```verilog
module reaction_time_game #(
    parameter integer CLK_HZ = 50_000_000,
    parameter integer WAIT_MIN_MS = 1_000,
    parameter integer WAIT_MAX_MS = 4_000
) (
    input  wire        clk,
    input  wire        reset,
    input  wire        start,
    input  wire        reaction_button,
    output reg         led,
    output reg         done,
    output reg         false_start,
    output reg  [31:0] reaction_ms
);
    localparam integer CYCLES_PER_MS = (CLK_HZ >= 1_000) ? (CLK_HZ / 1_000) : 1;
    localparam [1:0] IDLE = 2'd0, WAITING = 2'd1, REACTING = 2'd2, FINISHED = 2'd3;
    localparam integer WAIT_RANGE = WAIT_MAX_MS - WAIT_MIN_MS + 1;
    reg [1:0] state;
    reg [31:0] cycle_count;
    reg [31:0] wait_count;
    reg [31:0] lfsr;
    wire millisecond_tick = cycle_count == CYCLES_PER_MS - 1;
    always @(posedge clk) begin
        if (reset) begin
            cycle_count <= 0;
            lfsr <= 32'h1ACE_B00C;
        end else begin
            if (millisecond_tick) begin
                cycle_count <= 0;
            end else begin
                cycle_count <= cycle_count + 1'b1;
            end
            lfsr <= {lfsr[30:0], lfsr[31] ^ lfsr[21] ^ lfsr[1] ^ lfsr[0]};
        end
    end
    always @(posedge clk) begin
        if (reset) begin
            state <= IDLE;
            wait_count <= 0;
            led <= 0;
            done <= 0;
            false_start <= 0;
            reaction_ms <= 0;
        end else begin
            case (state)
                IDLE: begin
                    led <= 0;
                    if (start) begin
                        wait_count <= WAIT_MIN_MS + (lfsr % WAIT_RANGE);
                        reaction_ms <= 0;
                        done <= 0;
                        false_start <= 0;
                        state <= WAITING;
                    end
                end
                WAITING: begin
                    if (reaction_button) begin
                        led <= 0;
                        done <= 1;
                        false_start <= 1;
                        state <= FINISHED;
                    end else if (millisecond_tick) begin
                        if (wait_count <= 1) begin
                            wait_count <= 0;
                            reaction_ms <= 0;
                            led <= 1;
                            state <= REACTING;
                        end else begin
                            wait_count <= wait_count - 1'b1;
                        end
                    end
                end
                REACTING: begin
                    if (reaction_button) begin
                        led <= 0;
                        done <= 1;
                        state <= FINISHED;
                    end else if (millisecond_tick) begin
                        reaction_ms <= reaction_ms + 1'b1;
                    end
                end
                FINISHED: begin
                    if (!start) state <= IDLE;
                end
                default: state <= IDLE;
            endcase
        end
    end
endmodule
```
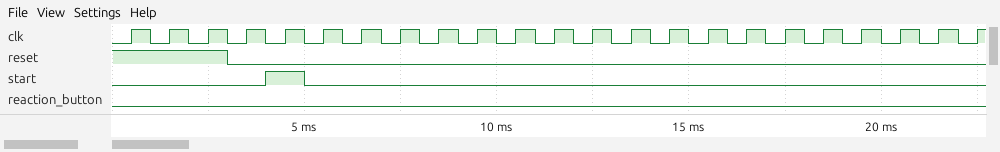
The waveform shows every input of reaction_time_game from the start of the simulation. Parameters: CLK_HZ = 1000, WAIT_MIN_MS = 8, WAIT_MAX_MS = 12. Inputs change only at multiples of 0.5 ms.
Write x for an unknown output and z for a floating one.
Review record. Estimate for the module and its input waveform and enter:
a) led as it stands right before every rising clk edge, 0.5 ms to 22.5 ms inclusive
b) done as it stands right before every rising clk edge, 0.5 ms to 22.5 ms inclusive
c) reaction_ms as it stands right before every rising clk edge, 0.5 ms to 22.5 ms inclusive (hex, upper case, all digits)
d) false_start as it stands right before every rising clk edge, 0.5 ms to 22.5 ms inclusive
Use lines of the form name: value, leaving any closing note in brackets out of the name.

led as it stands right before every rising clk edge, 0.5 ms to 22.5 ms inclusive: x 0 0 0 0 0 0 0 0 0 0 0 0 1 1 1 1 1 1 1 1 1 1
done as it stands right before every rising clk edge, 0.5 ms to 22.5 ms inclusive: x 0 0 0 0 0 0 0 0 0 0 0 0 0 0 0 0 0 0 0 0 0 0
reaction_ms as it stands right before every rising clk edge, 0.5 ms to 22.5 ms inclusive: x, 00000000, 00000000, 00000000, 00000000, 00000000, 00000000, 00000000, 00000000, 00000000, 00000000, 00000000, 00000000, 00000000, 00000001, 00000002, 00000003, 00000004, 00000005, 00000006, 00000007, 00000008, 00000009
false_start as it stands right before every rising clk edge, 0.5 ms to 22.5 ms inclusive: x 0 0 0 0 0 0 0 0 0 0 0 0 0 0 0 0 0 0 0 0 0 0
